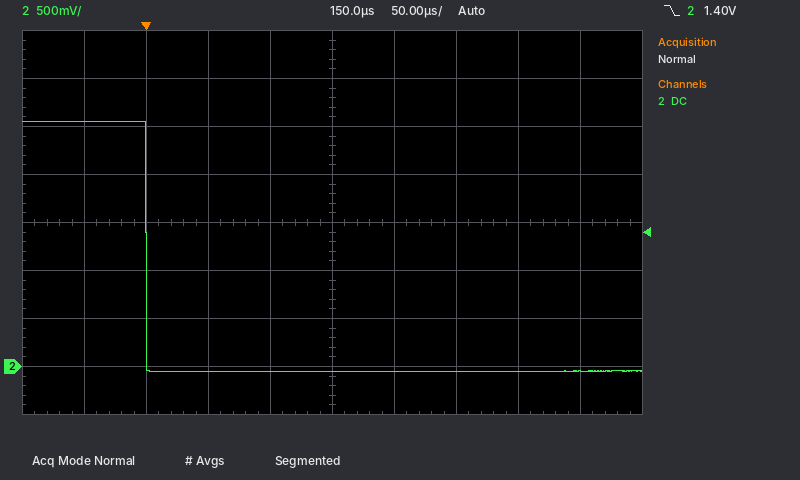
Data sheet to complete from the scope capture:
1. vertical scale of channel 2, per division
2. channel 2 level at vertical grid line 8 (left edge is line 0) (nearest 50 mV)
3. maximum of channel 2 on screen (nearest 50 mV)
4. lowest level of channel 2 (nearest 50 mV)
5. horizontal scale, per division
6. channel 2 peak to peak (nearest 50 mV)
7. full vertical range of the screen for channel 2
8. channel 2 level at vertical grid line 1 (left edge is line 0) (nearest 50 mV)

500 mV
-50 mV
2.55 V
-50 mV
50 µs
2.60 V
4 V
2.55 V
